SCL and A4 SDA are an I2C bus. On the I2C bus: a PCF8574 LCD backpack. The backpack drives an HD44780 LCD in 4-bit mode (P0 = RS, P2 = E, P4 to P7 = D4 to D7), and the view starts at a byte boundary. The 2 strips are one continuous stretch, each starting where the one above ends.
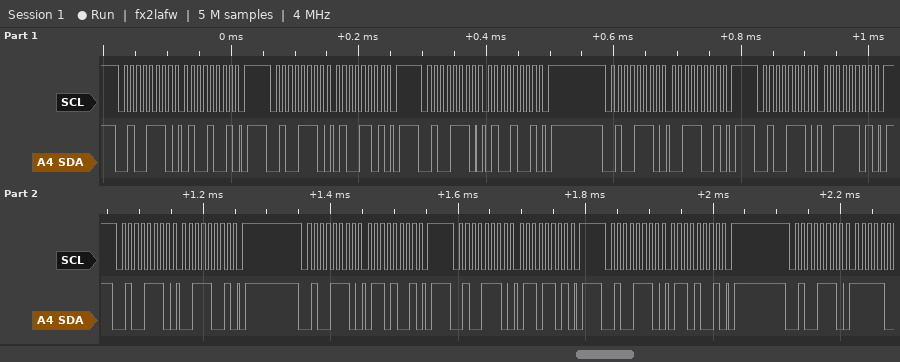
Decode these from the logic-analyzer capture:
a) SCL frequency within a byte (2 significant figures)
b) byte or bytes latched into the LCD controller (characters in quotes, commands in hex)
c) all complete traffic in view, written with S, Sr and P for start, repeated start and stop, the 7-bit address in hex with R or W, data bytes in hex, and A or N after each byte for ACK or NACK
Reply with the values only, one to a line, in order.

100 kHz
'C'
S 27W A 49 A P S 27W A 4D A P S 27W A 49 A P S 27W A 39 A P S 27W A 3D A P S 27W A 39 A P S 27W A 69 A P S 27W A 6D A P S 27W A 69 A P S 27W A
